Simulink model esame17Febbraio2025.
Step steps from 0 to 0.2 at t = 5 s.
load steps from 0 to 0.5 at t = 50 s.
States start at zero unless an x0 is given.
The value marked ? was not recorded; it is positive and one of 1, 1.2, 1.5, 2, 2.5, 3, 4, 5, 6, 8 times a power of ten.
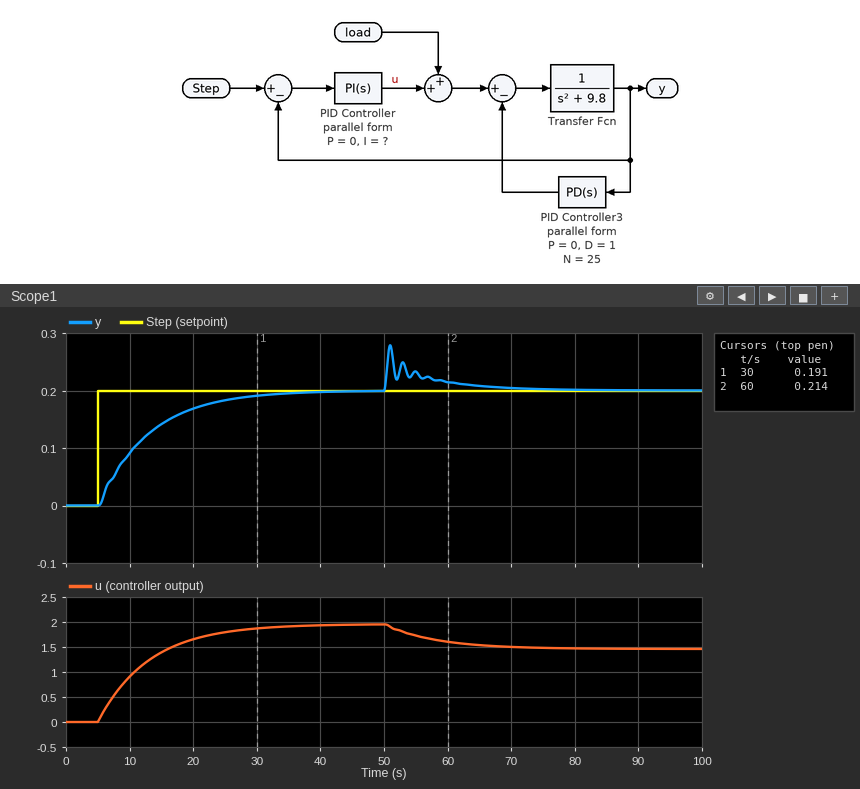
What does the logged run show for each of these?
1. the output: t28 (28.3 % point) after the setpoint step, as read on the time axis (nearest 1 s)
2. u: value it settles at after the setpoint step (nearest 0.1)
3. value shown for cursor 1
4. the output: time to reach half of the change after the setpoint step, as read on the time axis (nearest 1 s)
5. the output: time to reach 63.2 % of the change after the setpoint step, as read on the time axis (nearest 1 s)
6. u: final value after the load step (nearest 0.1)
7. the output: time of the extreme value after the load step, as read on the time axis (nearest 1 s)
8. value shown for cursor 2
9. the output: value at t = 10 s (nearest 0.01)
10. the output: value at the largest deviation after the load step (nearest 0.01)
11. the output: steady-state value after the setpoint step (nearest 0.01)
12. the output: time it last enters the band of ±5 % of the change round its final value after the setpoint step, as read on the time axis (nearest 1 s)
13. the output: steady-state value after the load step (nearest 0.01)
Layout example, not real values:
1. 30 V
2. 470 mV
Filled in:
1. 8 s
2. 2.0
3. 0.191
4. 11 s
5. 13 s
6. 1.5
7. 51 s
8. 0.214
9. 0.09
10. 0.28
11. 0.20
12. 29 s
13. 0.20
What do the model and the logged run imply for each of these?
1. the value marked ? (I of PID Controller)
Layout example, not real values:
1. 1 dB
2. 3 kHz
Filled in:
1. 1.2
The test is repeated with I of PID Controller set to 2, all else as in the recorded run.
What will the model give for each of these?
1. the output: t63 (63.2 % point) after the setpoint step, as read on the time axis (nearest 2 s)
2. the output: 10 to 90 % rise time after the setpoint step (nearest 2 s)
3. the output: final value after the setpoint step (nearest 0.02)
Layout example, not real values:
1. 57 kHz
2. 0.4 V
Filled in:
1. 10 s
2. 10 s
3. 0.20
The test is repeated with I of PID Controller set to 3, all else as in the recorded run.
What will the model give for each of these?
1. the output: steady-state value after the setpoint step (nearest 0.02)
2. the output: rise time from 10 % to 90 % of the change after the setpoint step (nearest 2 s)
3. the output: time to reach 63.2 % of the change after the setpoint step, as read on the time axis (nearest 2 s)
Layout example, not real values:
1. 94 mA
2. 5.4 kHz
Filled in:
1. 0.20
2. 6 s
3. 8 s
